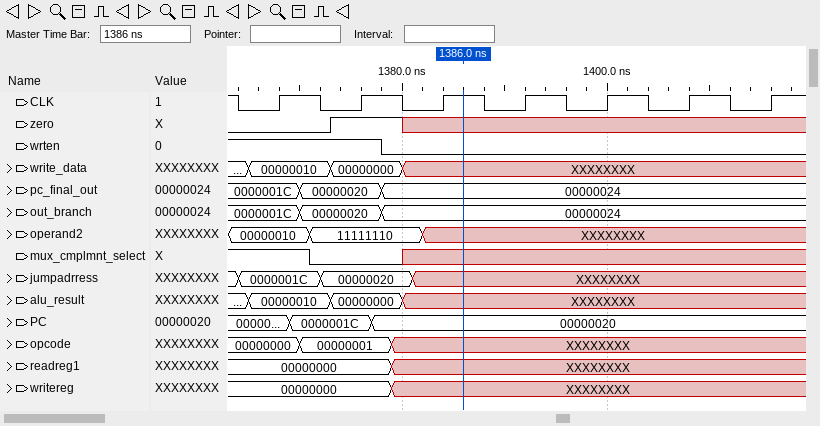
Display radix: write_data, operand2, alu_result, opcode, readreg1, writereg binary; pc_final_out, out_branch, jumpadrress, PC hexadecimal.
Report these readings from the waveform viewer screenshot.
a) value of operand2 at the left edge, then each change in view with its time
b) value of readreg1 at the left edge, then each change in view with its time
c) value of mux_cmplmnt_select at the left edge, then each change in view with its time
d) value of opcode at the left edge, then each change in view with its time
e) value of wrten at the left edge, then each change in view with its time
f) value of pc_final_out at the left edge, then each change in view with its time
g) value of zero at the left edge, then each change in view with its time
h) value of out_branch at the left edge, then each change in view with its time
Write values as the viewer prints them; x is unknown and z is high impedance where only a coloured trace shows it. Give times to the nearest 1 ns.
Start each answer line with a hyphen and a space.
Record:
- 00000010, 11111110 at 1371 ns, XXXXXXXX at 1382 ns
- 00000000, XXXXXXXX at 1379 ns
- 1, 0 at 1371 ns, x at 1380 ns
- 00000000, 00000001 at 1370 ns, XXXXXXXX at 1379 ns
- 1, 0 at 1378 ns
- 0000001C, 00000020 at 1370 ns, 00000024 at 1378 ns
- 0, 1 at 1373 ns, x at 1380 ns
- 0000001C, 00000020 at 1370 ns, 00000024 at 1378 ns
